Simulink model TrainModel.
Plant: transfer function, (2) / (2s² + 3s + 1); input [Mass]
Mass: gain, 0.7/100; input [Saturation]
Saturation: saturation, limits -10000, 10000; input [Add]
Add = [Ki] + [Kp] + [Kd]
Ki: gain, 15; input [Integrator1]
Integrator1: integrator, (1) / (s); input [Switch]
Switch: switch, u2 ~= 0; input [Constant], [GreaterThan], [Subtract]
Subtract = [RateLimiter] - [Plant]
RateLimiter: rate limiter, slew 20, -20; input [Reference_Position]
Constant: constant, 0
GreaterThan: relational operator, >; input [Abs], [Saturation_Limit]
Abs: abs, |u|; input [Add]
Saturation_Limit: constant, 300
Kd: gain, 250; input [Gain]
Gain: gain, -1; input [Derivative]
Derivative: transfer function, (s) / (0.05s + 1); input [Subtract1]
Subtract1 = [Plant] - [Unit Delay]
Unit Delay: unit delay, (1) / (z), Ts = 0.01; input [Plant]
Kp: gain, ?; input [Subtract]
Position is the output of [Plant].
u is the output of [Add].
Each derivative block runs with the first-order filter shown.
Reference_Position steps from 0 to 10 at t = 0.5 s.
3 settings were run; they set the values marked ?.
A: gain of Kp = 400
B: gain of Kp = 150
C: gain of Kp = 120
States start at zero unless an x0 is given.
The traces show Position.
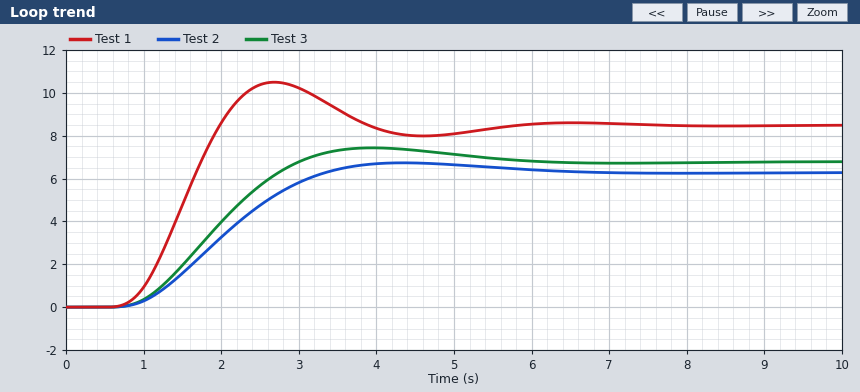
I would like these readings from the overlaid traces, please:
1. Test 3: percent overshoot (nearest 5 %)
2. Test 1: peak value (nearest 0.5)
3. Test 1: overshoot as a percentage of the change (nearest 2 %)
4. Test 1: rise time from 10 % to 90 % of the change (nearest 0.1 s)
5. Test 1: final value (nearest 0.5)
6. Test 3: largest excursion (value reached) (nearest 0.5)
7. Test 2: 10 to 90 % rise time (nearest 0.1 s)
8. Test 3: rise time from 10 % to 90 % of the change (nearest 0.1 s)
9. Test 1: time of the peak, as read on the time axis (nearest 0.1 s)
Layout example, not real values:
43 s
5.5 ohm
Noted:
10 %
10.5
24 %
0.9 s
8.5
7.5
1.7 s
1.5 s
2.7 s
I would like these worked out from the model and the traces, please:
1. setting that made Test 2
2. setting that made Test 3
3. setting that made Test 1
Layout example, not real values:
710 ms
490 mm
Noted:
C
B
A
